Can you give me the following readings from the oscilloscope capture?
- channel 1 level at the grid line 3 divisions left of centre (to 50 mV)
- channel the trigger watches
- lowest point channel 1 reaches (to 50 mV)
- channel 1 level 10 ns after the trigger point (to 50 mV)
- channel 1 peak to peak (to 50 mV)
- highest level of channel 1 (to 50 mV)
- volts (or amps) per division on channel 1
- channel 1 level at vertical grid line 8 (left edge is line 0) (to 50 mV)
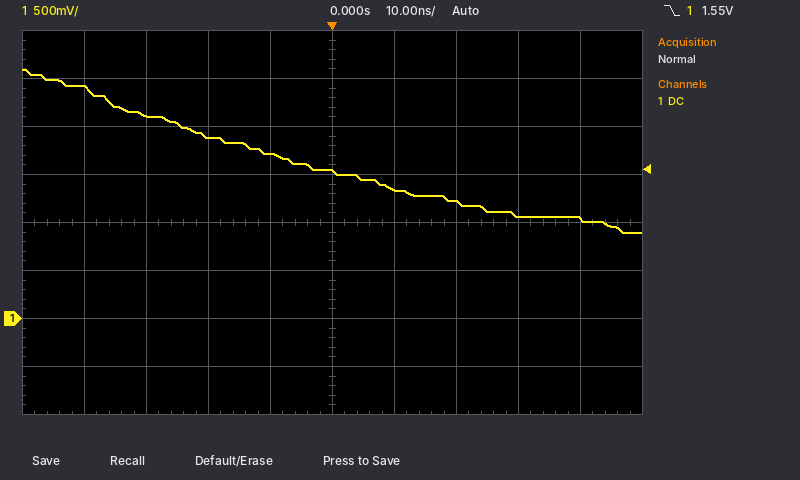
2.10 V
channel 1
900 mV
1.35 V
1.70 V
2.60 V
500 mV
1.05 V
